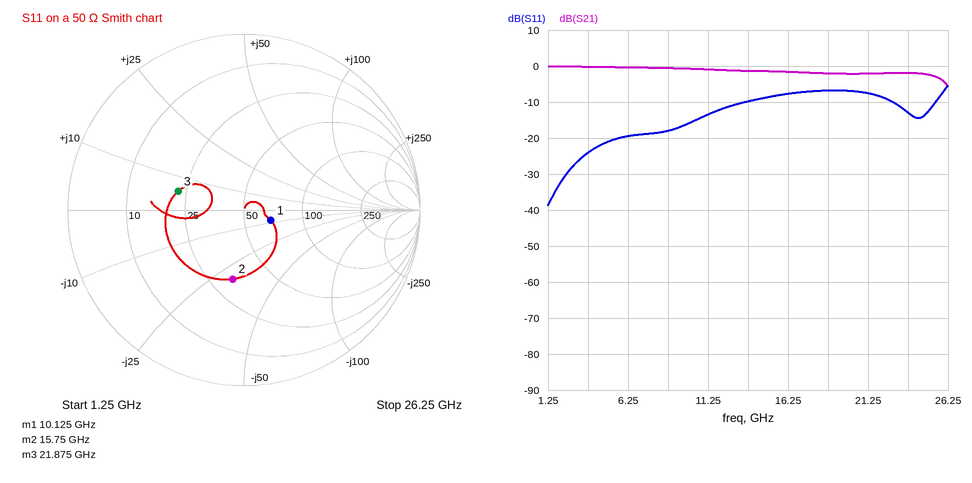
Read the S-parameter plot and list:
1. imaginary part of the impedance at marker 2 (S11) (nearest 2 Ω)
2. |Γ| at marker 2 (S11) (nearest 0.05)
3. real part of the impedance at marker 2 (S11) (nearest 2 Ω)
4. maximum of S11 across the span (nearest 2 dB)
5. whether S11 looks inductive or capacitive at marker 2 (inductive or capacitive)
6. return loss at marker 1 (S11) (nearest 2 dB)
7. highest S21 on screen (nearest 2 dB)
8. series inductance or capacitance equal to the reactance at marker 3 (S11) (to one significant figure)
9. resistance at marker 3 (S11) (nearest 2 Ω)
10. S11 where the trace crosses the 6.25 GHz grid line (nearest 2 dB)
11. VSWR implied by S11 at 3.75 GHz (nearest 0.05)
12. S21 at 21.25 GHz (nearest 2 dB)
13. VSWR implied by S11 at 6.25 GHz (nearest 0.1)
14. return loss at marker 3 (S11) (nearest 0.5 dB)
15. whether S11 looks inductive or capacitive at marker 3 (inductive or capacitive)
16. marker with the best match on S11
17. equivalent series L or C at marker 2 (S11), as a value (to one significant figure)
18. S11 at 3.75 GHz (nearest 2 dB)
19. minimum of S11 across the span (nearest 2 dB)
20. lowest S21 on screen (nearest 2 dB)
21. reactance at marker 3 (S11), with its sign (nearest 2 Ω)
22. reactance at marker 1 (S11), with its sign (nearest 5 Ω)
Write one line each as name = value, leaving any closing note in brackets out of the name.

imaginary part of the impedance at marker 2 (S11) = -30 Ω
|Γ| at marker 2 (S11) = 0.40
real part of the impedance at marker 2 (S11) = 32 Ω
maximum of S11 across the span = -6 dB
whether S11 looks inductive or capacitive at marker 2 = capacitive
return loss at marker 1 (S11) = 16 dB
highest S21 on screen = 0 dB
series inductance or capacitance equal to the reactance at marker 3 (S11) = 40 pH
resistance at marker 3 (S11) = 22 Ω
S11 where the trace crosses the 6.25 GHz grid line = -20 dB
VSWR implied by S11 at 3.75 GHz = 1.15
S21 at 21.25 GHz = -2 dB
VSWR implied by S11 at 6.25 GHz = 1.2
return loss at marker 3 (S11) = 8.0 dB
whether S11 looks inductive or capacitive at marker 3 = inductive
marker with the best match on S11 = marker 1
equivalent series L or C at marker 2 (S11), as a value = 300 fF
S11 at 3.75 GHz = -24 dB
minimum of S11 across the span = -38 dB
lowest S21 on screen = -6 dB
reactance at marker 3 (S11), with its sign = +6 Ω
reactance at marker 1 (S11), with its sign = -10 Ω
